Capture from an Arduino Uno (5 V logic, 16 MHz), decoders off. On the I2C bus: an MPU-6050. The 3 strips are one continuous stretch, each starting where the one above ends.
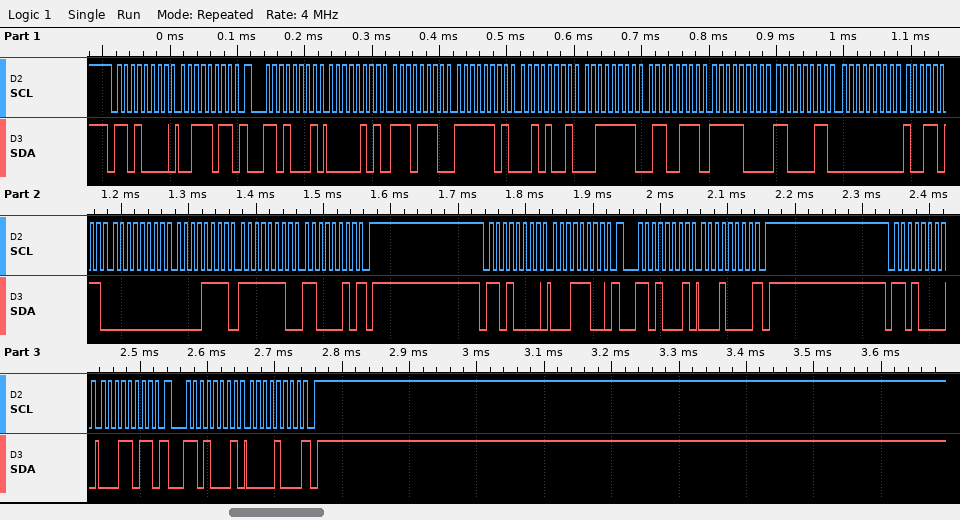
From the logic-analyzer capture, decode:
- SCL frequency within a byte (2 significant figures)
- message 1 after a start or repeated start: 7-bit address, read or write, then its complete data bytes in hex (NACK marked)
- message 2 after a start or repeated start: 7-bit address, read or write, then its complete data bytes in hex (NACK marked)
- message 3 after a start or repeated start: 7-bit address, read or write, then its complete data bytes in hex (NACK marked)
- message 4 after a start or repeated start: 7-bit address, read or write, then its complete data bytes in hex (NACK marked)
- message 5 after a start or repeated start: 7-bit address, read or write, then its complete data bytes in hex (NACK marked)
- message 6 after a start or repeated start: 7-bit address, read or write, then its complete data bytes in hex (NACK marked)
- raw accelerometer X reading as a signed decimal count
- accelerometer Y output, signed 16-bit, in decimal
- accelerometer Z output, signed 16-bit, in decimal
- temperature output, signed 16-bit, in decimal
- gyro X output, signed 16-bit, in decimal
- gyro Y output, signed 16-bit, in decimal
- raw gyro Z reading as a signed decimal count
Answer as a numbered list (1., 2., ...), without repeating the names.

1. 100 kHz
2. 0x68 write: 3B
3. 0x68 read: 05 EE FD 29 3F 67 F8 C3 00 9B 00 0F FE C2 NACK
4. 0x68 write: 1C
5. 0x68 read: 10 NACK
6. 0x68 write: 1B
7. 0x68 read: 08 NACK
8. 1518
9. -727
10. 16231
11. -1853
12. 155
13. 15
14. -318
